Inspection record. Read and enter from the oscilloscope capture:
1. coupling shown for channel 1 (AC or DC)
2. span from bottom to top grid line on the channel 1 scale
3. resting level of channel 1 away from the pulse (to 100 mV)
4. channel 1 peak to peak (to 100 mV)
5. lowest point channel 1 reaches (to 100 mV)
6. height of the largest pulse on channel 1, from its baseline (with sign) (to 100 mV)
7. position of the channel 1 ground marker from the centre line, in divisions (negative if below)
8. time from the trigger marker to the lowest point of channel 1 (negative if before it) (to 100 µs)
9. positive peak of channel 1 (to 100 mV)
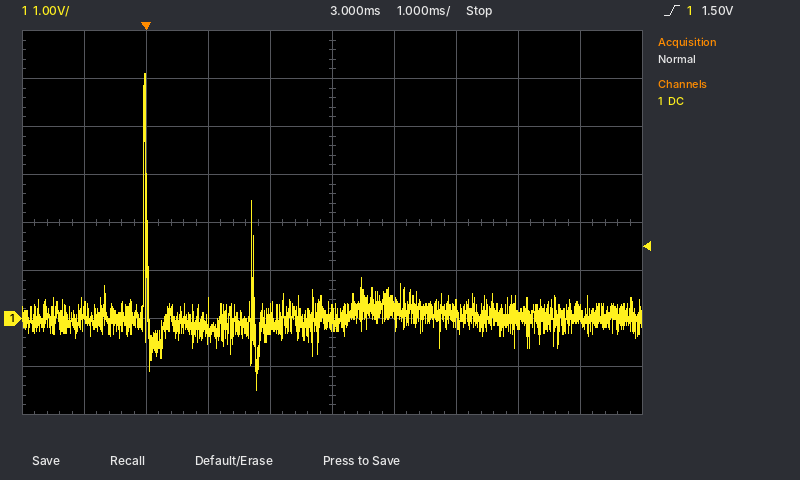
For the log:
DC
8 V
0.0 V
6.6 V
-1.5 V
+5.1 V
-2.0 div
+1.8 ms
5.1 V
